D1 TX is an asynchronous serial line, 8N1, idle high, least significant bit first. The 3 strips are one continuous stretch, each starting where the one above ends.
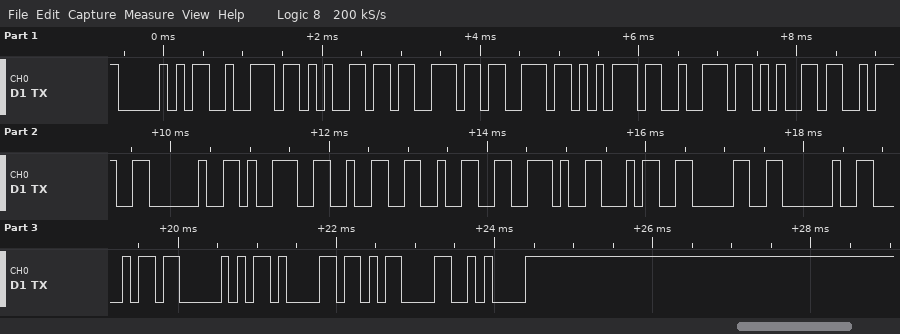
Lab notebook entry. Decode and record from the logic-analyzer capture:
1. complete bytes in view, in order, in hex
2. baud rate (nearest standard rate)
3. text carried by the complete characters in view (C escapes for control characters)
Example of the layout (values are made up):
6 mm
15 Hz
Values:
50 72 65 73 73 75 72 65 3A 20 39 32 32 2E 34 30 20 68 50 61 0D 0A
9600 baud
"Pressure: 922.40 hPa\r\n"
